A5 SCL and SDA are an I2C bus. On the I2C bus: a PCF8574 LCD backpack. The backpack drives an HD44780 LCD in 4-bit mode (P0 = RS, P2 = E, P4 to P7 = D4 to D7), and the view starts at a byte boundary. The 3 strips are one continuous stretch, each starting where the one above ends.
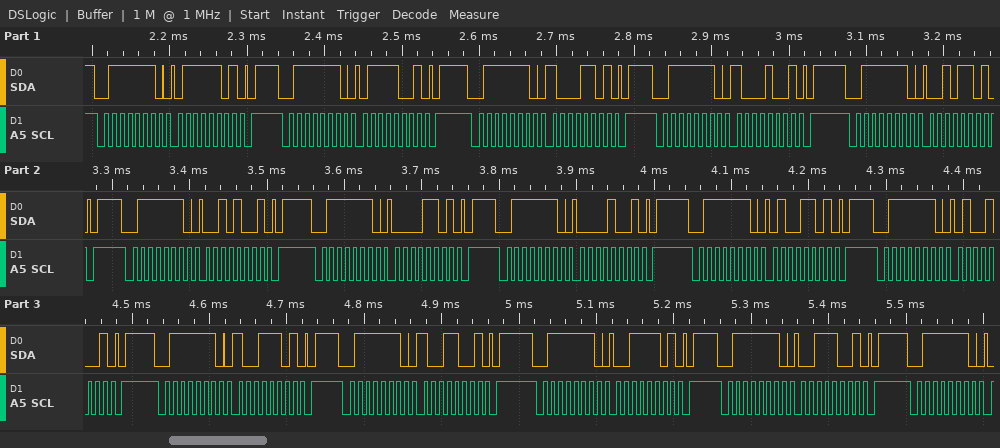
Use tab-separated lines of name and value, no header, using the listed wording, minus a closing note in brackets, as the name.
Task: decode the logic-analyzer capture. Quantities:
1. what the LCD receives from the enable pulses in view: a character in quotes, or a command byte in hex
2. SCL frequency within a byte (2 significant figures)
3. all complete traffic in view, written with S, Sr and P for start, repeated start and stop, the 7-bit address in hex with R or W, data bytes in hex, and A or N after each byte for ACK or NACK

what the LCD receives from the enable pulses in view: a character in quotes, or a command byte in hex	'x' ' ' 'I'
SCL frequency within a byte	100 kHz
all complete traffic in view, written with S, Sr and P for start, repeated start and stop, the 7-bit address in hex with R or W, data bytes in hex, and A or N after each byte for ACK or NACK	S 3FW A 7D A P S 3FW A 79 A P S 3FW A 8D A P S 3FW A 89 A P S 3FW A 2D A P S 3FW A 29 A P S 3FW A 0D A P S 3FW A 09 A P S 3FW A 4D A P S 3FW A 49 A P S 3FW A 9D A P S 3FW A 99 A P S 3FW A 3D A P S 3FW A 39 A P S 3FW A
